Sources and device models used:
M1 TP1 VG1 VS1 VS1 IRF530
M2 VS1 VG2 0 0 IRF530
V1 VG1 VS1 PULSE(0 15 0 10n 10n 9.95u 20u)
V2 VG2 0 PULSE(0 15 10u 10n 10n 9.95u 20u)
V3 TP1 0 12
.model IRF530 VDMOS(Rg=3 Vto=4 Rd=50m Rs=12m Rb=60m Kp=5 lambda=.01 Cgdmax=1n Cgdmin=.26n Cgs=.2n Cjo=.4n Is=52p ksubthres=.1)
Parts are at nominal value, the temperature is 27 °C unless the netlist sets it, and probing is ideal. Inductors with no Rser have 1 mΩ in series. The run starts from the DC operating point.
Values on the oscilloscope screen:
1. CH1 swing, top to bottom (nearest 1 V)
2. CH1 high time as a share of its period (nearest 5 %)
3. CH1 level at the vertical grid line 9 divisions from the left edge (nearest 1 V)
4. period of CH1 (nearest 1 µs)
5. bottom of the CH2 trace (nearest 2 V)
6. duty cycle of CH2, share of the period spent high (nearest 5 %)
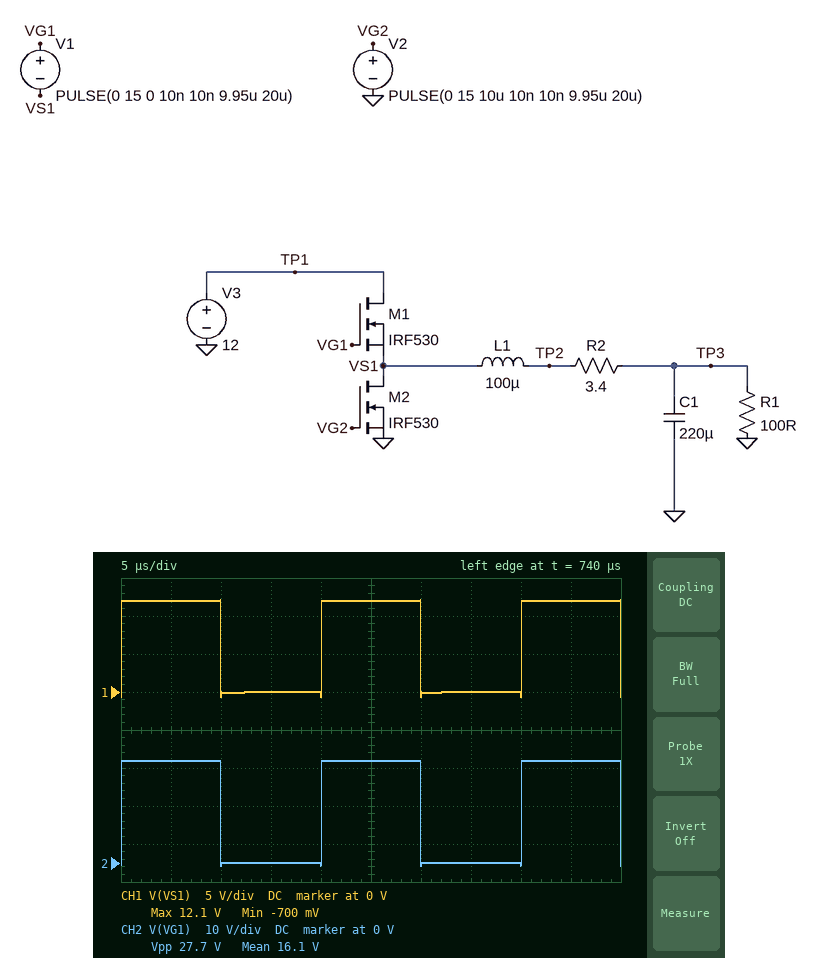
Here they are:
13 V
50 %
12 V
20 µs
0 V
50 %
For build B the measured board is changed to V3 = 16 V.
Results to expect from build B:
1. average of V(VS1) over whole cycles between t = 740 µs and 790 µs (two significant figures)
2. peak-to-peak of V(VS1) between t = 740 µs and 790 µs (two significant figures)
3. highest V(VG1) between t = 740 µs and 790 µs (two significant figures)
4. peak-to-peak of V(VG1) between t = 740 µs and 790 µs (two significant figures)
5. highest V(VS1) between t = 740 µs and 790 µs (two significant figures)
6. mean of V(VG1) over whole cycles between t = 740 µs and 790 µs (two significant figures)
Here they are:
7.9 V
17 V
31 V
32 V
16 V
15 V
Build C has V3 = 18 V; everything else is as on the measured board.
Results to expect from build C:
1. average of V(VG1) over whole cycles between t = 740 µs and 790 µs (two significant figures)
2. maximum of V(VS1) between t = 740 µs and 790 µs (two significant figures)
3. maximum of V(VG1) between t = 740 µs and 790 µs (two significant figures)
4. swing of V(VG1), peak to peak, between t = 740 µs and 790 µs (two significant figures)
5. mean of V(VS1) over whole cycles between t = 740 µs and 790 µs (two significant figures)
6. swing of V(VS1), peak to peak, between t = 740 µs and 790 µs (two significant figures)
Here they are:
16 V
18 V
33 V
34 V
8.9 V
19 V
